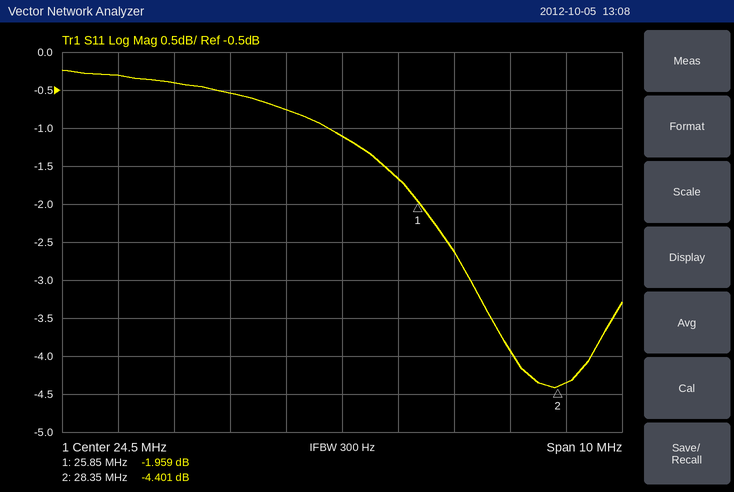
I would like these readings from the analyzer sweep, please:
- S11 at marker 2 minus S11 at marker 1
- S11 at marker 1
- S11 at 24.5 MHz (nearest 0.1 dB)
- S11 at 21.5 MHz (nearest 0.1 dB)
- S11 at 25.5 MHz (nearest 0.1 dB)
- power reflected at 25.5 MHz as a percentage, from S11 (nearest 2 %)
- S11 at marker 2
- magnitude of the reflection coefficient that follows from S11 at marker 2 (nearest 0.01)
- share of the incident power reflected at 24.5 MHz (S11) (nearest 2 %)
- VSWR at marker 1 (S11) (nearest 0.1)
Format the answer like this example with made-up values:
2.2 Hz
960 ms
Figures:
-2.442 dB
-1.959 dB
-1.1 dB
-0.4 dB
-1.7 dB
68 %
-4.401 dB
0.60
78 %
8.9
